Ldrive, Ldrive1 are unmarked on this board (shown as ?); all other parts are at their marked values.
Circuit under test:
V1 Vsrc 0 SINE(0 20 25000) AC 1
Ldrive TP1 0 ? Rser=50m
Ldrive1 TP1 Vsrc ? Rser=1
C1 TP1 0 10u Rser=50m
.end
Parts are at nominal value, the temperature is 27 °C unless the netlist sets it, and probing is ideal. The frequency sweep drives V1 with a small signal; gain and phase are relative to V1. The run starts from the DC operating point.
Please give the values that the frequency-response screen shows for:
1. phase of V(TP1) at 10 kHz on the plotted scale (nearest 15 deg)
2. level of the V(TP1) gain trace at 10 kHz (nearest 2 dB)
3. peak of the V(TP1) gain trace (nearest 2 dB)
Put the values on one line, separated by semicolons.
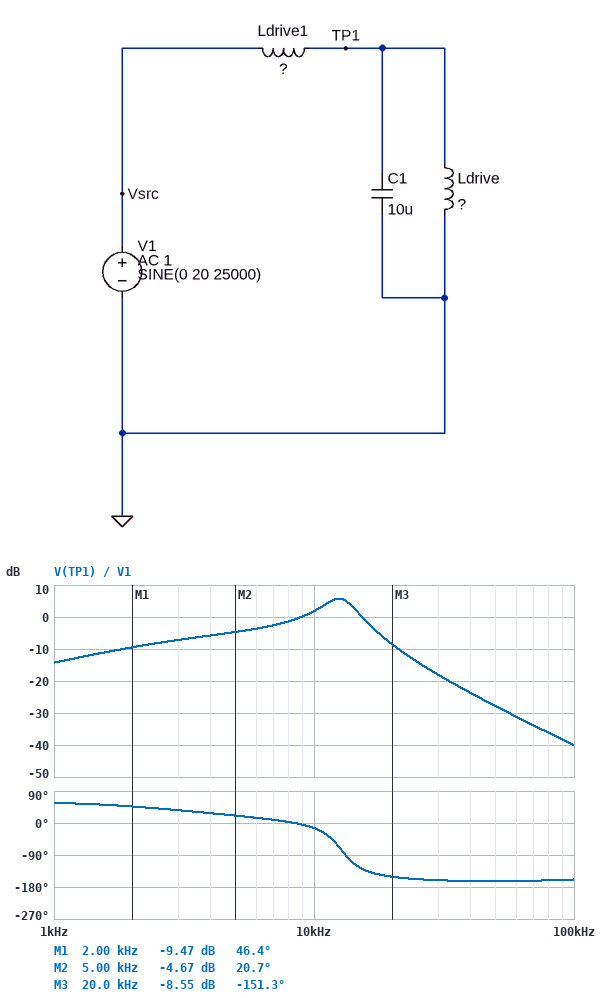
-15 deg; 2 dB; 6 dB
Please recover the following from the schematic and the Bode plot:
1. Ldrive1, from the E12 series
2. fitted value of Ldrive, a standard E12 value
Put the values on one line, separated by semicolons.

27 µH; 33 µH
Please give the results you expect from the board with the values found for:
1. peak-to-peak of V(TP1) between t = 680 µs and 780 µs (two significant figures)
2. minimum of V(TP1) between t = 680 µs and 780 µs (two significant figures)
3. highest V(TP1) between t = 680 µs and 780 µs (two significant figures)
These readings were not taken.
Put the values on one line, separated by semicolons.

7.9 V; -4.0 V; 4.0 V
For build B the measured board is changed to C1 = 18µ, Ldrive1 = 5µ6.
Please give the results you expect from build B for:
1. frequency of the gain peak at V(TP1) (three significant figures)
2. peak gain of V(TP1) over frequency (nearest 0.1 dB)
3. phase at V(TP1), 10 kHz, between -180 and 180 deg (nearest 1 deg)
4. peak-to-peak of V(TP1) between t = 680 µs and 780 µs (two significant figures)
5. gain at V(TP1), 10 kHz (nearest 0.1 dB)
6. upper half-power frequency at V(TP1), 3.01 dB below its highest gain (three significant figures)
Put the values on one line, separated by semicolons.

7.85 kHz; -0.2 dB; -38 deg; 13 V; -0.7 dB; 14.5 kHz
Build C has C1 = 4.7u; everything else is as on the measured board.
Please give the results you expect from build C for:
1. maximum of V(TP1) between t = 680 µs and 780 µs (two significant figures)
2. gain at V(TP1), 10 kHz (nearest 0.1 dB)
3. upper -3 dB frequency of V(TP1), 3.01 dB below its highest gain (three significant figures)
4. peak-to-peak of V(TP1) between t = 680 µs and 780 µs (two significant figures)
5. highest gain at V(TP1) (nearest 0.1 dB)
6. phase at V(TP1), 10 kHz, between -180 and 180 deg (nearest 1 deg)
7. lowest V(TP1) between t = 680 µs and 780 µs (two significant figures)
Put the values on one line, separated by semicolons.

14 V; -2.6 dB; 20.5 kHz; 28 V; 8.8 dB; 7 deg; -14 V
